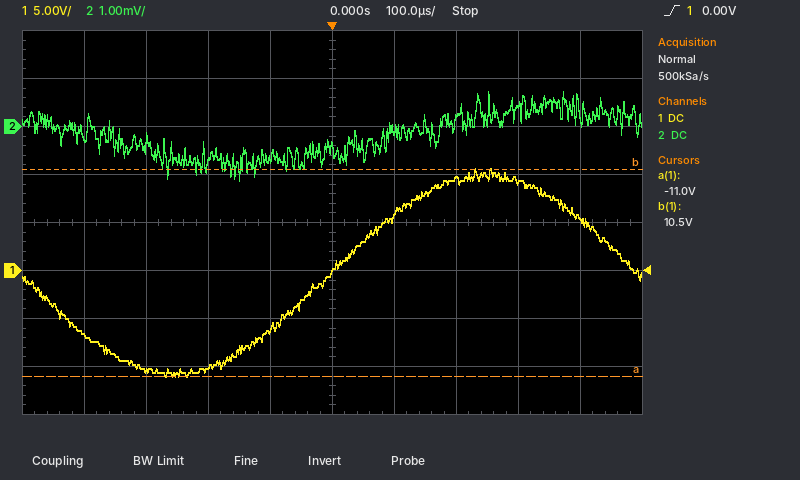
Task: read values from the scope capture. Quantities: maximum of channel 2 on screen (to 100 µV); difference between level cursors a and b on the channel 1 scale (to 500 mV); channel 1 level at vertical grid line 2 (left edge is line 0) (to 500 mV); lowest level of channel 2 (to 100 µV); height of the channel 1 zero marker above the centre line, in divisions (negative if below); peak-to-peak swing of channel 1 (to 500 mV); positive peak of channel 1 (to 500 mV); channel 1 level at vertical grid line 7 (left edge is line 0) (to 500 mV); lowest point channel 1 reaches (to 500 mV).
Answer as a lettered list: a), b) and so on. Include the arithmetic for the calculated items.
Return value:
a) 700 µV
b) 21.5 V
c) -10.5 V
d) -1.1 mV
e) -1.0 div
f) 10.5 V − (-11.0 V) = 21.5 V
g) 10.5 V
h) 9.5 V
i) -11.0 V
